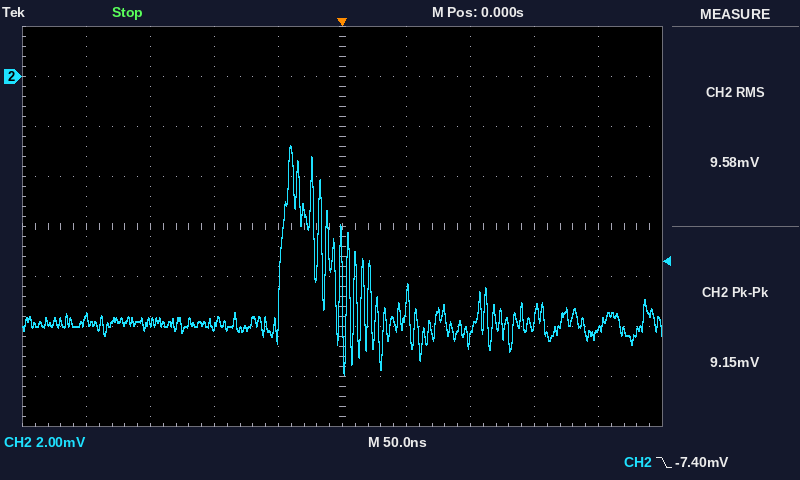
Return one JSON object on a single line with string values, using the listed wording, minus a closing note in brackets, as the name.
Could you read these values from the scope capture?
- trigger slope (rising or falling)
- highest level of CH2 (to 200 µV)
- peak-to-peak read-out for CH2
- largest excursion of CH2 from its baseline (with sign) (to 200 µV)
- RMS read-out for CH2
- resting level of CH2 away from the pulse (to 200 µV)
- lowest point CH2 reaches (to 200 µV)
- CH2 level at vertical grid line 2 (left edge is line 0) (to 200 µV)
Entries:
{"trigger slope": "falling", "highest level of CH2": "-2.8 mV", "peak-to-peak read-out for CH2": "9.15 mV", "largest excursion of CH2 from its baseline (with sign)": "+7.0 mV", "RMS read-out for CH2": "9.58 mV", "resting level of CH2 away from the pulse": "-9.8 mV", "lowest point CH2 reaches": "-12.0 mV", "CH2 level at vertical grid line 2 (left edge is line 0)": "-9.8 mV"}
